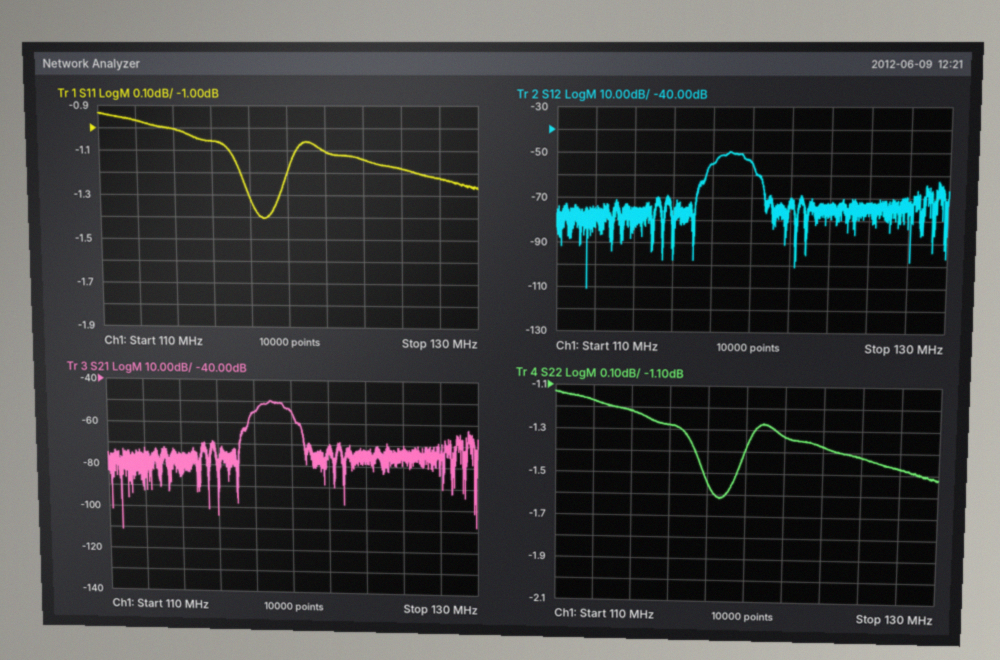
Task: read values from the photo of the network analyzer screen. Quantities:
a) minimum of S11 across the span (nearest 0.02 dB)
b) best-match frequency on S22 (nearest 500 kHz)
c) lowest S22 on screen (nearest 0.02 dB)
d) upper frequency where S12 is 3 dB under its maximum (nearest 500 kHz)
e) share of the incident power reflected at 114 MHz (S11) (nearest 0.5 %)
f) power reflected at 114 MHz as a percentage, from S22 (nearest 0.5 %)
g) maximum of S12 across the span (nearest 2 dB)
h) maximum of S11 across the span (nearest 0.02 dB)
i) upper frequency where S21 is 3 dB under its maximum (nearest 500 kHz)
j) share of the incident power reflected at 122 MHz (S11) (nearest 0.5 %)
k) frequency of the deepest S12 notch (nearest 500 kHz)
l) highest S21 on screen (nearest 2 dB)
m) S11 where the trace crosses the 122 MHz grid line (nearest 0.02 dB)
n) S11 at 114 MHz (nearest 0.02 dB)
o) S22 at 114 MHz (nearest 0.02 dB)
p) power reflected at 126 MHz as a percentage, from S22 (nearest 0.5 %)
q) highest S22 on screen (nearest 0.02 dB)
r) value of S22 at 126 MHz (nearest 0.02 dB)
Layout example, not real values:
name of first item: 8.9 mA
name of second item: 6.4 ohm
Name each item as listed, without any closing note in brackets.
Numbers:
minimum of S11 across the span: -1.40 dB
best-match frequency on S22: 118.5 MHz
lowest S22 on screen: -1.62 dB
upper frequency where S12 is 3 dB under its maximum: 119.5 MHz
share of the incident power reflected at 114 MHz (S11): 79.5 %
power reflected at 114 MHz as a percentage, from S22: 75.5 %
maximum of S12 across the span: -50 dB
maximum of S11 across the span: -0.94 dB
upper frequency where S21 is 3 dB under its maximum: 119.5 MHz
share of the incident power reflected at 122 MHz (S11): 77.5 %
frequency of the deepest S12 notch: 111.5 MHz
highest S21 on screen: -50 dB
S11 where the trace crosses the 122 MHz grid line: -1.10 dB
S11 at 114 MHz: -1.00 dB
S22 at 114 MHz: -1.22 dB
power reflected at 126 MHz as a percentage, from S22: 72.0 %
highest S22 on screen: -1.12 dB
value of S22 at 126 MHz: -1.42 dB
